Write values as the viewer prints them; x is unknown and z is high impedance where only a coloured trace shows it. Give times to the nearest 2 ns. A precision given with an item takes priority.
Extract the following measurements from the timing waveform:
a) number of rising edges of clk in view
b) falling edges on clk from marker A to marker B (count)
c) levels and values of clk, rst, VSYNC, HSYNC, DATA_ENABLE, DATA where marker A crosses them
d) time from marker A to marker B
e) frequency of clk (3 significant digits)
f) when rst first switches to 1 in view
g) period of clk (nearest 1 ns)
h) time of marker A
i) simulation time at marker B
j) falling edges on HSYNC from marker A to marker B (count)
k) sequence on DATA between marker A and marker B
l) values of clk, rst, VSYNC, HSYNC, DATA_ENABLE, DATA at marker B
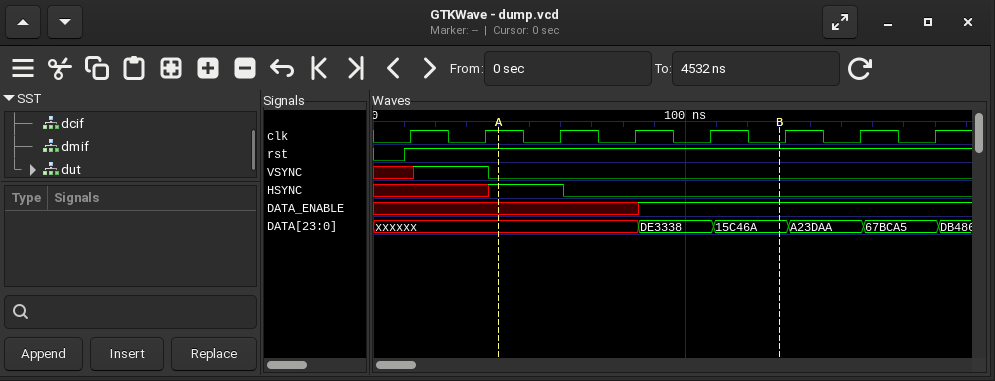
8
4
clk=1, rst=1, VSYNC=0, HSYNC=1, DATA_ENABLE=x, DATA=xxxxxx
90 ns
41.7 MHz
10 ns
24 ns
40 ns
130 ns
1
xxxxxx, DE3338, 15C46A
clk=0, rst=1, VSYNC=0, HSYNC=0, DATA_ENABLE=1, DATA=15C46A
